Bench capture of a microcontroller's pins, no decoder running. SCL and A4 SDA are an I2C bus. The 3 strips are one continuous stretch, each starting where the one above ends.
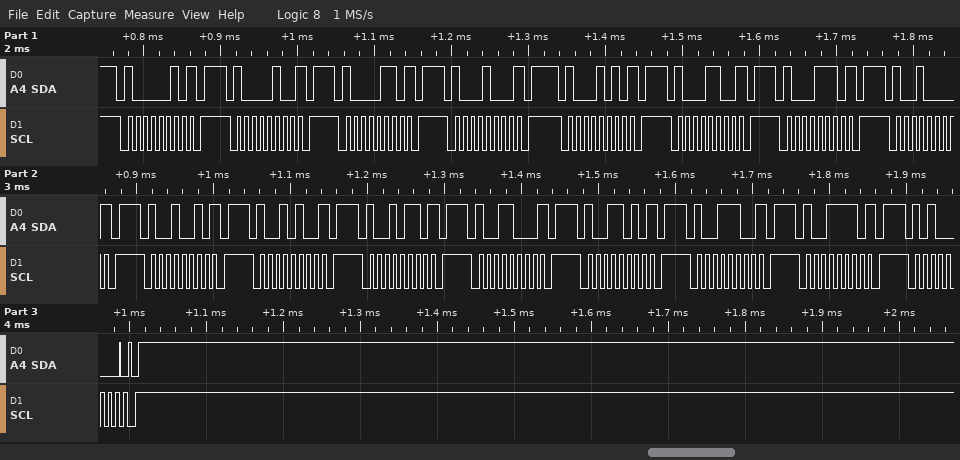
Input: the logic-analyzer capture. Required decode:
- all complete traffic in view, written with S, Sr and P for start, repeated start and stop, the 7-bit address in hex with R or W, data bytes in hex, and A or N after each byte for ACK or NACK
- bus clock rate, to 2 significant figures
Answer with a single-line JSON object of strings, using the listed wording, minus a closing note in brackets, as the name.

{"all complete traffic in view, written with S, Sr and P for start, repeated start and stop, the 7-bit address in hex with R or W, data bytes in hex, and A or N after each byte for ACK or NACK": "S 41W N P S 42W N P S 43W N P S 44W N P S 45W N P S 46W N P S 47W N P S 48W N P S 49W N P S 4AW N P S 4BW N P S 4CW N P S 4DW N P S 4EW N P S 4FW N P S 50W A P", "bus clock rate, to 2 significant figures": "100 kHz"}
